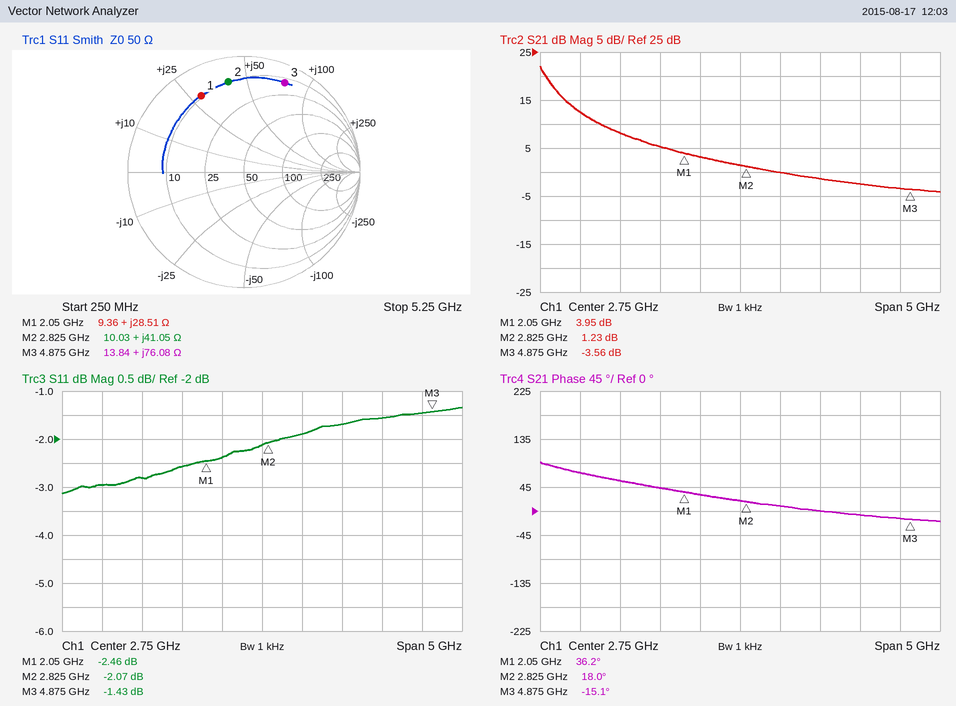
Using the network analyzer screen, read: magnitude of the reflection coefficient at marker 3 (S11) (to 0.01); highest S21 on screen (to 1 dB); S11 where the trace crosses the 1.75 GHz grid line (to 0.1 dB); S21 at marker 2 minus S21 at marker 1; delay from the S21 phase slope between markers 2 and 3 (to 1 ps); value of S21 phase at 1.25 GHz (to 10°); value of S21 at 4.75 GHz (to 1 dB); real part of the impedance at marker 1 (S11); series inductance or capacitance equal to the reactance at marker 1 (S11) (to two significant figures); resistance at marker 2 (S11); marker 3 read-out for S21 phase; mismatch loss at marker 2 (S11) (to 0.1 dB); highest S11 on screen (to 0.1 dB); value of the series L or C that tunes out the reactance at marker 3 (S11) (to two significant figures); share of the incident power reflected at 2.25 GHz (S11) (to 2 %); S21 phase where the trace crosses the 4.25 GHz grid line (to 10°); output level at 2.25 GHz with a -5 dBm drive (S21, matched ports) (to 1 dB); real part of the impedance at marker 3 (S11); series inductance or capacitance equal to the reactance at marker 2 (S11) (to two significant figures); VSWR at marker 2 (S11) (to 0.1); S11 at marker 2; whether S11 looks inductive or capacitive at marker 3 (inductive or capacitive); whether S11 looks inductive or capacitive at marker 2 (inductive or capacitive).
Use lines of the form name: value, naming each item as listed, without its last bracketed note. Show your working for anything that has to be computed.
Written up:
magnitude of the reflection coefficient at marker 3 (S11): 0.85
highest S21 on screen: 22 dB
S11 where the trace crosses the 1.75 GHz grid line: -2.6 dB
S21 at marker 2 minus S21 at marker 1: 1.23 − (3.95) = -2.72 dB
delay from the S21 phase slope between markers 2 and 3: −(-15.1° − (18°))/(360° × 2.05 GHz) ≈ 45 ps
value of S21 phase at 1.25 GHz: 60°
value of S21 at 4.75 GHz: -3 dB
real part of the impedance at marker 1: 9.36 Ω
series inductance or capacitance equal to the reactance at marker 1 (S11): L = 28.51 Ω/(2π × 2.05 GHz) ≈ 2.2 nH
resistance at marker 2: 10.03 Ω
marker 3 read-out for S21 phase: -15.1°
mismatch loss at marker 2 (S11): −10 log10(1 − 10^(-2.07/10)) ≈ 4.2 dB
highest S11 on screen: -1.3 dB
value of the series L or C that tunes out the reactance at marker 3 (S11): C = 1/(2π × 4.875 GHz × 76.08 Ω) ≈ 429 fF, so 430 fF to two significant figures
share of the incident power reflected at 2.25 GHz (S11): 10^(-2.4/10) ≈ 58 %
S21 phase where the trace crosses the 4.25 GHz grid line: -10°
output level at 2.25 GHz with a -5 dBm drive (S21, matched ports): -5 dBm + (3 dB) = -2 dBm
real part of the impedance at marker 3: 13.84 Ω
series inductance or capacitance equal to the reactance at marker 2 (S11): L = 41.05 Ω/(2π × 2.825 GHz) ≈ 2.3 nH
VSWR at marker 2 (S11): 8.4
S11 at marker 2: -2.07 dB
whether S11 looks inductive or capacitive at marker 3: inductive
whether S11 looks inductive or capacitive at marker 2: inductive
